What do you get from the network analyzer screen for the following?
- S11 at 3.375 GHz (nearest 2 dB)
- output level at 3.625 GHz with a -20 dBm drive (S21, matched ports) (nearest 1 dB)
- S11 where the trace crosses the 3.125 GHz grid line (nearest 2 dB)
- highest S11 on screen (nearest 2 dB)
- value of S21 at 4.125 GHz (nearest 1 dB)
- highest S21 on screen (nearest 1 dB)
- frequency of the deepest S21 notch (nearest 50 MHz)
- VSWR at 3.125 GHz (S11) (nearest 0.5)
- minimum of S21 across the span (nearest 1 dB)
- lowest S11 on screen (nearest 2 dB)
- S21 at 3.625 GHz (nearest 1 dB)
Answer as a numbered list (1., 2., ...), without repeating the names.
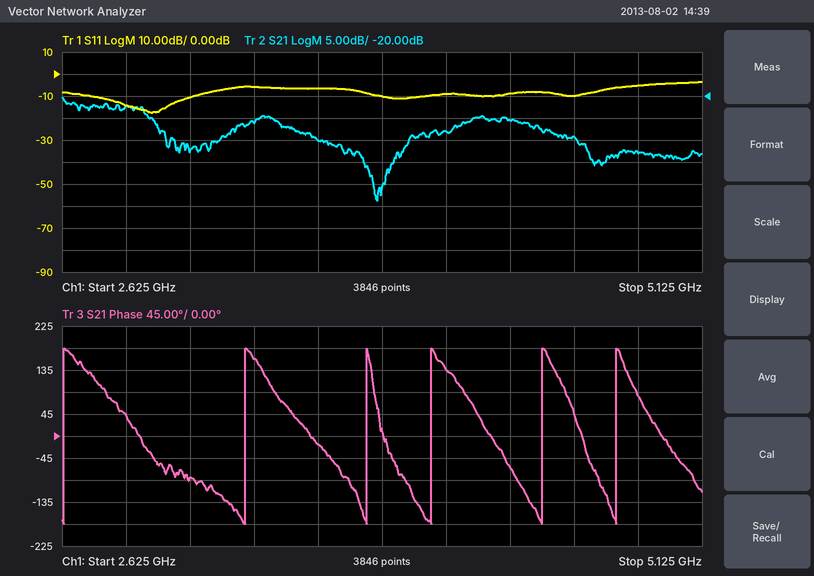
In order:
1. -6 dB
2. -50 dBm
3. -10 dB
4. -4 dB
5. -28 dB
6. -20 dB
7. 3.85 GHz
8. 2.0
9. -44 dB
10. -18 dB
11. -30 dB
